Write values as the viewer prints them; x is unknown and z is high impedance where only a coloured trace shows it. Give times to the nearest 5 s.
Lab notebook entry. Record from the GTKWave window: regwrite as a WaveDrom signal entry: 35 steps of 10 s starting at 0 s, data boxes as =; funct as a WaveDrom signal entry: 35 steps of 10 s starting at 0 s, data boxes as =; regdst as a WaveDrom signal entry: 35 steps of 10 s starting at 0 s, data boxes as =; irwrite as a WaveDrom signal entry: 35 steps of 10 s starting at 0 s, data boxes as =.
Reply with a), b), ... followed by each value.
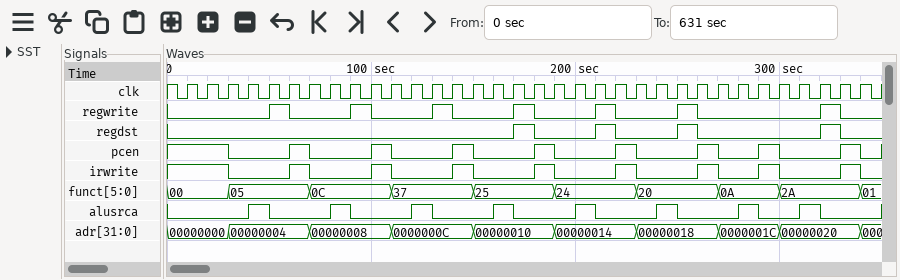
a) {name: 'regwrite', wave: '0....10..10..10..10..10..10.....10.'}
b) {name: 'funct', wave: '=..=...=...=...=...=...=...=..=...=', data: '00 05 0C 37 25 24 20 0A 2A 01'}
c) {name: 'regdst', wave: '0................10..10..10.....10.'}
d) {name: 'irwrite', wave: '1..0..10..10..10..10..10..10.10..10'}
